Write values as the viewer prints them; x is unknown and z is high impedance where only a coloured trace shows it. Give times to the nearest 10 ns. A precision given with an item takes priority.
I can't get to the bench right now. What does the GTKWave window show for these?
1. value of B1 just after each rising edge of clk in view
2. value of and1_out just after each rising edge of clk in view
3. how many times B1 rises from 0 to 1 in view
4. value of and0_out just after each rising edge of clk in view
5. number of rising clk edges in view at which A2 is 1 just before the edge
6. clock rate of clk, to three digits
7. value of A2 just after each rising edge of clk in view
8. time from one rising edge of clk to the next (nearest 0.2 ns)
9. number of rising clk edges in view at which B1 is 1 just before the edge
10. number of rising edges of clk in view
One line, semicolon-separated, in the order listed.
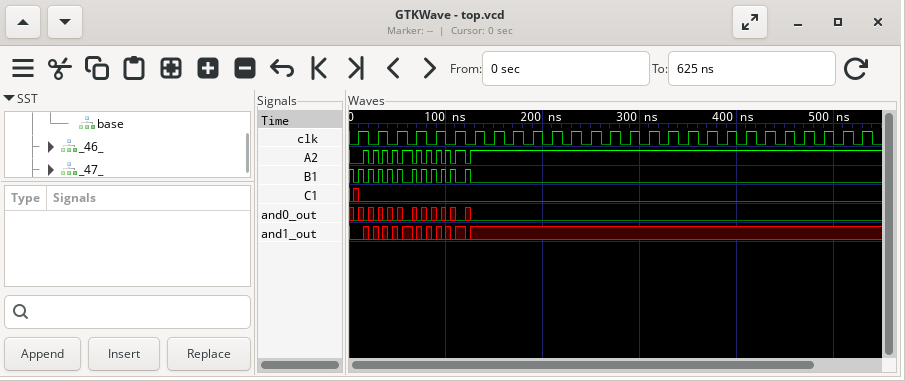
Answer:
1 1 1 0 0 0 0 0 0 0 0 0 0 0 0 0 0 0 0 0 0 0 0 0 0 0 0; 0 0 0 x x x x x x x x x x x x x x x x x x x x x x x x; 11; x x x 0 0 0 0 0 0 0 0 0 0 0 0 0 0 0 0 0 0 0 0 0 0 0 0; 23; 50.0 MHz; 0 0 0 1 1 1 1 1 1 1 1 1 1 1 1 1 1 1 1 1 1 1 1 1 1 1 1; 20 ns; 3; 27
